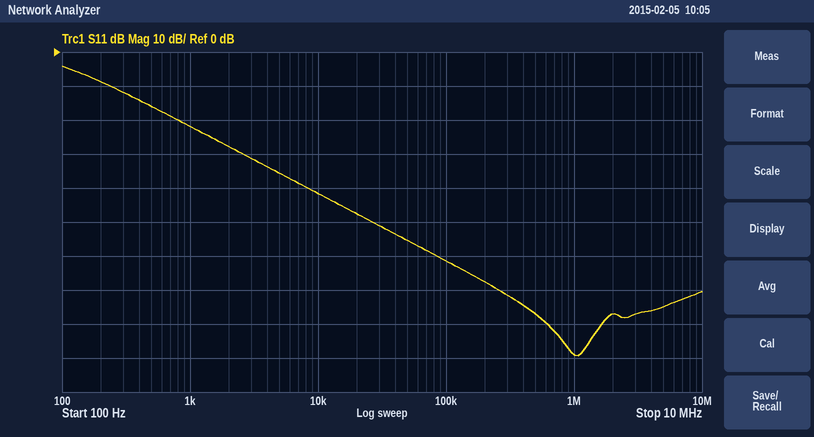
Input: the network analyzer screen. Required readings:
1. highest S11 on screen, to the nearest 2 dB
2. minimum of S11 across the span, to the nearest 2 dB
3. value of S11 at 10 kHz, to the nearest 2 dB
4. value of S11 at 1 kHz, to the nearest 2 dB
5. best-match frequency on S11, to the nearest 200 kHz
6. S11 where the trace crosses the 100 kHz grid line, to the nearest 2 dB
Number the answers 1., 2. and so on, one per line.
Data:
1. -4 dB
2. -90 dB
3. -42 dB
4. -22 dB
5. 1.0 MHz
6. -62 dB
